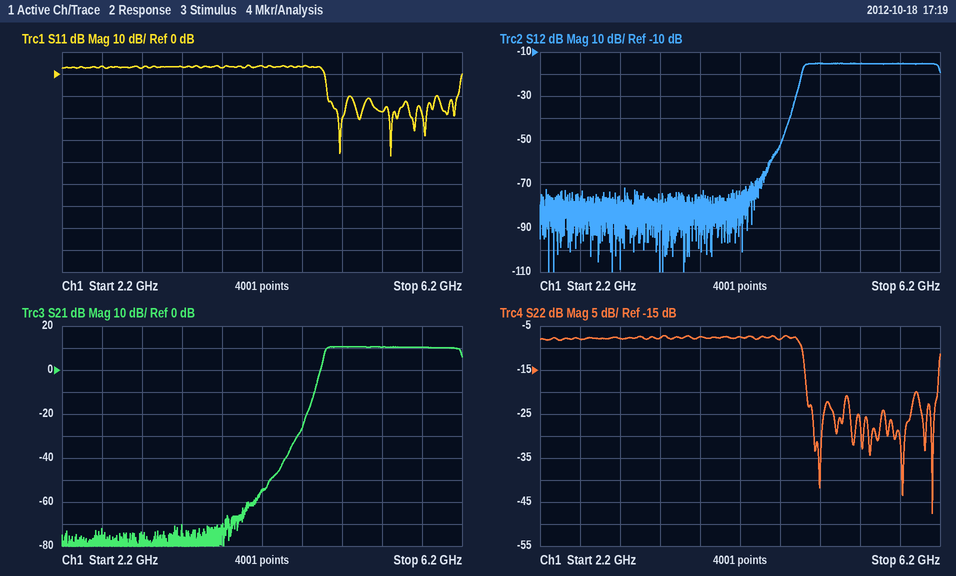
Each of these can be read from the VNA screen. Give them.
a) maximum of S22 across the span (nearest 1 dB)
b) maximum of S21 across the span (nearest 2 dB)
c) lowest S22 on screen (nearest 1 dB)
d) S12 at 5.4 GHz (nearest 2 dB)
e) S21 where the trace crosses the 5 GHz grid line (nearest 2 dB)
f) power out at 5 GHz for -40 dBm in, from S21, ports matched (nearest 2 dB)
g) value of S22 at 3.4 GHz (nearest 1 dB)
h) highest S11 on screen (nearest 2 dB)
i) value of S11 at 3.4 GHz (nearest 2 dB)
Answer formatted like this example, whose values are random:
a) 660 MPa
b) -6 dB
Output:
a) -7 dB
b) 10 dB
c) -48 dB
d) -16 dB
e) 10 dB
f) -30 dBm
g) -8 dB
h) 4 dB
i) 4 dB
